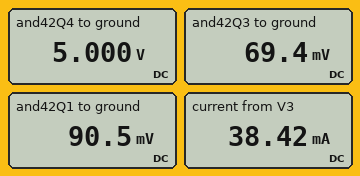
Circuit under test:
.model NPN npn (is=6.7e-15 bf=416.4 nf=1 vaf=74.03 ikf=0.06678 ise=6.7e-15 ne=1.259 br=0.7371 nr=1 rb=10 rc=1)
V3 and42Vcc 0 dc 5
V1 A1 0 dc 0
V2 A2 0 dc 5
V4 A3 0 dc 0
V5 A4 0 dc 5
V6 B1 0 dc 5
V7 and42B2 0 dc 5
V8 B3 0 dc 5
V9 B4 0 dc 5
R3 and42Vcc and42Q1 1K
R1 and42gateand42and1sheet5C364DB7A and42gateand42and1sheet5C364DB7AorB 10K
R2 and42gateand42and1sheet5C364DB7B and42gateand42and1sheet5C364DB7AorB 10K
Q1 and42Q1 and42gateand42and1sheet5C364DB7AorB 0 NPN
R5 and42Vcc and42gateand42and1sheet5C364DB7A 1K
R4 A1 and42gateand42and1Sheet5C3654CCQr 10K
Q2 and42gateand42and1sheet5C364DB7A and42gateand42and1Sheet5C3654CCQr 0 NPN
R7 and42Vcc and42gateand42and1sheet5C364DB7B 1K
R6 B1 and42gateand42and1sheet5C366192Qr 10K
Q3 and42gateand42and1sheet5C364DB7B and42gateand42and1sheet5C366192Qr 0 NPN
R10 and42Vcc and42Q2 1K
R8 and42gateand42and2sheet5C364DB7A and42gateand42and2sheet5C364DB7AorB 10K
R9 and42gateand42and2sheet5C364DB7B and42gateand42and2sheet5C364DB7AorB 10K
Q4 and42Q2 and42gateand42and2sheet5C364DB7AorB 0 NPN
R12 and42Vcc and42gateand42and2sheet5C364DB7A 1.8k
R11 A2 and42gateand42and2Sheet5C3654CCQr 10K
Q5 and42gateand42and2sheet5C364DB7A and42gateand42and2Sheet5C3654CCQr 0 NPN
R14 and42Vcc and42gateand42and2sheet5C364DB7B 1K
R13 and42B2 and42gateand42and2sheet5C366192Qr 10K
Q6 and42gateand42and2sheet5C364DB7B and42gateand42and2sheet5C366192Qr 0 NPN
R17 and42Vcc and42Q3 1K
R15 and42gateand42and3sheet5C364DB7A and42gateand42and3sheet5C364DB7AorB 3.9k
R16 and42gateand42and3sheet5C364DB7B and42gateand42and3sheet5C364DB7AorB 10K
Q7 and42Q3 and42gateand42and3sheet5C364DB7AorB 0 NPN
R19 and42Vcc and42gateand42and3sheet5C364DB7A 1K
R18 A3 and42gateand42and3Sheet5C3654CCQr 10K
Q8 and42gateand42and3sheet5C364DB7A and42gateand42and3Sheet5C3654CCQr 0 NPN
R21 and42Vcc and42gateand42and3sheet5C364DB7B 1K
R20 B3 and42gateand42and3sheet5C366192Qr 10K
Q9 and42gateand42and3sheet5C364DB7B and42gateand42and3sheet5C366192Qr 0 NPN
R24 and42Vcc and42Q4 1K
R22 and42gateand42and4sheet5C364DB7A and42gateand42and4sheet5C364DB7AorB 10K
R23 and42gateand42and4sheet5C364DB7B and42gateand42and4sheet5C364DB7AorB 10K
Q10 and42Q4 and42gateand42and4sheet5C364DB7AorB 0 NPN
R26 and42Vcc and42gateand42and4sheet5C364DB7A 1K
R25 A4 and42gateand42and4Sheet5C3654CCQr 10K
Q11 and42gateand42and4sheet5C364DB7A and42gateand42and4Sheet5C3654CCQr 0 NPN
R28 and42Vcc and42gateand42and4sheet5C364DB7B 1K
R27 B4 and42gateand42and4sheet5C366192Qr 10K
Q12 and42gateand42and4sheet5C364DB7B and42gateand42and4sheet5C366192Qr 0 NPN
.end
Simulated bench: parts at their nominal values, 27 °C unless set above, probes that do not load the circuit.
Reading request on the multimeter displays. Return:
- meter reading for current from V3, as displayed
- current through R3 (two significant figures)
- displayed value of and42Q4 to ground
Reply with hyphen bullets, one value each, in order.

- 38.42 mA
- 4.9 mA
- 5.000 V
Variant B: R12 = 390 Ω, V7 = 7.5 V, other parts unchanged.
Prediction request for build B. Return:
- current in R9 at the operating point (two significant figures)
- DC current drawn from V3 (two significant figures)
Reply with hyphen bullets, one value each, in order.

- 2.3 µA
- 48 mA
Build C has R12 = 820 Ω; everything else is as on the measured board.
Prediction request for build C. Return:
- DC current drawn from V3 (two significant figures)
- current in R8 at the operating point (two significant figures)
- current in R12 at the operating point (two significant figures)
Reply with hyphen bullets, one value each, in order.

- 42 mA
- 320 nA
- 6.0 mA
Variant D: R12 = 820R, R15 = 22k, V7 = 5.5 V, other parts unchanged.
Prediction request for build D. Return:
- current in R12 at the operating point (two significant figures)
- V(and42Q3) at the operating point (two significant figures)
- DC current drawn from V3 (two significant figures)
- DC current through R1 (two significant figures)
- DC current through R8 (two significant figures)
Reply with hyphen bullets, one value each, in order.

- 6.0 mA
- 120 mV
- 41 mA
- 390 µA
- 450 nA
